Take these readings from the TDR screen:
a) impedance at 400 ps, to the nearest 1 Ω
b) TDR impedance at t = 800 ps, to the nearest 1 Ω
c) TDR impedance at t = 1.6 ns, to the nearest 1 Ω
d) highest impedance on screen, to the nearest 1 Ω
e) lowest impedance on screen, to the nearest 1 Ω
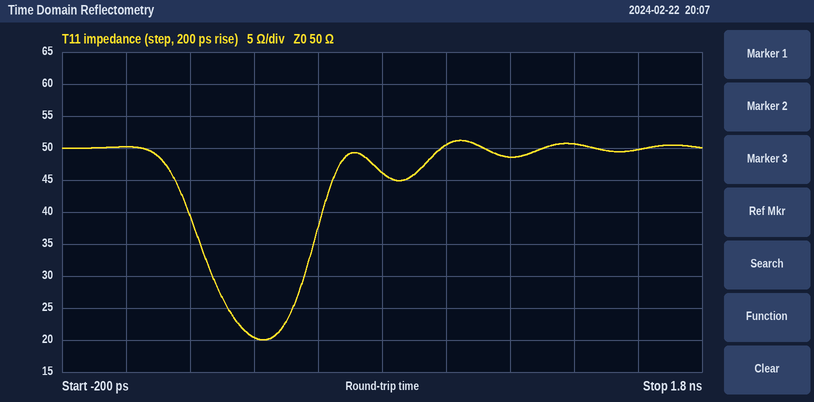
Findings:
20 Ω
46 Ω
50 Ω
51 Ω
20 Ω
